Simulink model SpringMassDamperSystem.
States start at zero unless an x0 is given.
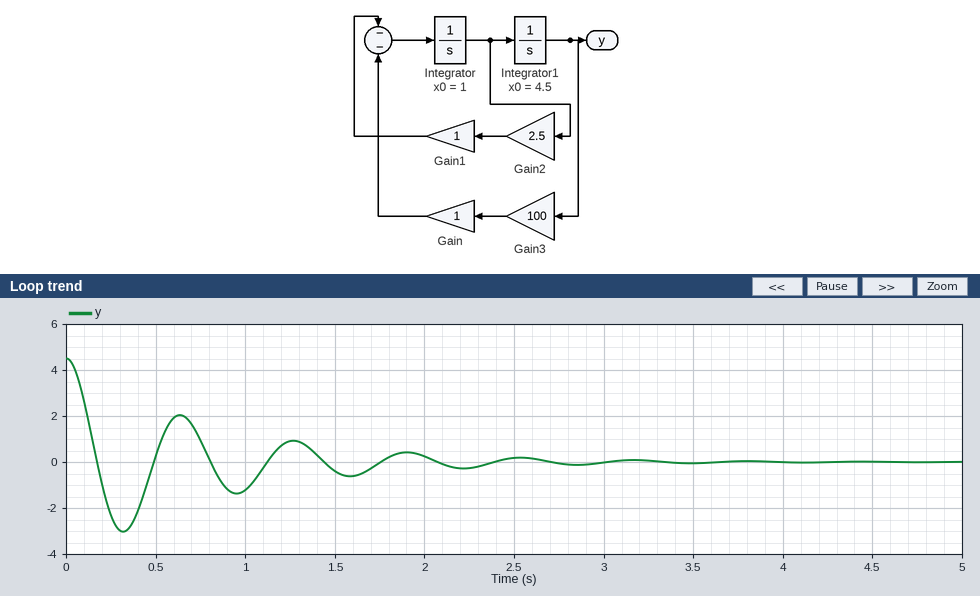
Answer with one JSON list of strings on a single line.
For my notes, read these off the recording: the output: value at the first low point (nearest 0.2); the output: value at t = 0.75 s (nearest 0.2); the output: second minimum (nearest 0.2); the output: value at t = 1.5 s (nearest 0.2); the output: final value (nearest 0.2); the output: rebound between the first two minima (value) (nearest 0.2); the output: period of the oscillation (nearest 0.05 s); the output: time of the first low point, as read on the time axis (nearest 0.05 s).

["-3.0", "1.0", "-1.4", "-0.4", "0.0", "2.0", "0.65 s", "0.30 s"]
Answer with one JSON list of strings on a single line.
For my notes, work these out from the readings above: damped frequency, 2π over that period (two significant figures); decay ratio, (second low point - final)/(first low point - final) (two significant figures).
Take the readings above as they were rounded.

["9.7 rad/s", "0.47"]
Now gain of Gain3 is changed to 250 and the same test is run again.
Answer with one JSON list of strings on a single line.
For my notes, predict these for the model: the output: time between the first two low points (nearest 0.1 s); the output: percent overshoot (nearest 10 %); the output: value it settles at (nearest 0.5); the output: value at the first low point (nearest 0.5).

["0.4 s", "80 %", "0.0", "-3.5"]
